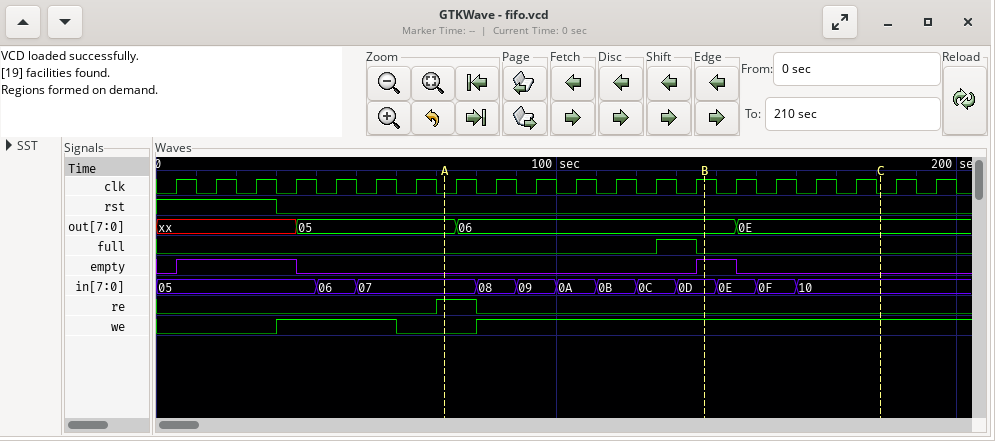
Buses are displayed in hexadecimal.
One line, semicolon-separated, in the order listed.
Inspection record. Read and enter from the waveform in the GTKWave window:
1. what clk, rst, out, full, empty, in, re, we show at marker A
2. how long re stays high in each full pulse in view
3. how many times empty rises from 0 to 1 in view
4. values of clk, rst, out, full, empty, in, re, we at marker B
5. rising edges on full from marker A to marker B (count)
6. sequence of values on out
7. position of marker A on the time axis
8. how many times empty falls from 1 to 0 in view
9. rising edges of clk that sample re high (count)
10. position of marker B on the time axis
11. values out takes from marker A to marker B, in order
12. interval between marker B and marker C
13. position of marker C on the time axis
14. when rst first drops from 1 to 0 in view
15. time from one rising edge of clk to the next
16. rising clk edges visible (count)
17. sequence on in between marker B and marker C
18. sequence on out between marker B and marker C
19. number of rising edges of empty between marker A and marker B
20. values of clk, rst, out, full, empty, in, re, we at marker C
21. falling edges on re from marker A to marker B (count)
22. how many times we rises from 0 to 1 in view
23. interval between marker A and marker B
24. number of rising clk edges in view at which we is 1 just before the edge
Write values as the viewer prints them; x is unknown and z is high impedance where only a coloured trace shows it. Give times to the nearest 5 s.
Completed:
clk=0, rst=0, out=05, full=0, empty=0, in=07, re=1, we=0; 10 s; 2; clk=1, rst=0, out=06, full=0, empty=1, in=0D, re=0, we=1; 1; xx, 05, 06, 0E; 70 s; 2; 1; 135 s; 05, 06; 45 s; 180 s; 30 s; 10 s; 20; 0D, 0E, 0F, 10; 06, 0E; 1; clk=0, rst=0, out=0E, full=0, empty=0, in=10, re=0, we=1; 1; 2; 65 s; 15
